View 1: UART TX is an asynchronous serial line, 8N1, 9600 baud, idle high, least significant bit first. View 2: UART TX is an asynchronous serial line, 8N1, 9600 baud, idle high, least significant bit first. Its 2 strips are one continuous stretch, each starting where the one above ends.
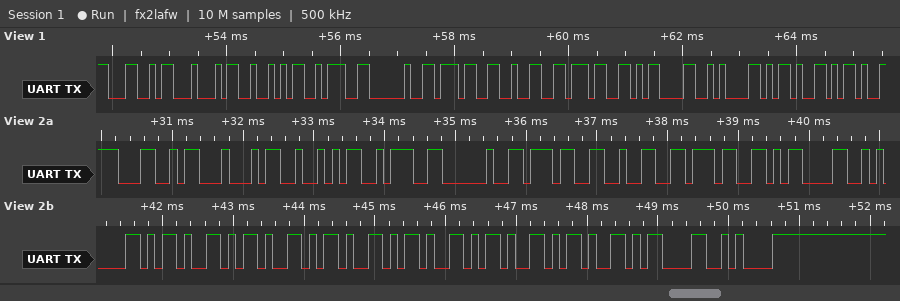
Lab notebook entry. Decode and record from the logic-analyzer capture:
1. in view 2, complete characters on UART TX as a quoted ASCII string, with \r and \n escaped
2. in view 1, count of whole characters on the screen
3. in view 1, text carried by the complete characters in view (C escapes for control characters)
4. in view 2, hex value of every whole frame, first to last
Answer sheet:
"LDR: 727\r\n------\r\n"
12
"LDR: 727\r\n--"
4C 44 52 3A 20 37 32 37 0D 0A 2D 2D 2D 2D 2D 2D 0D 0A
